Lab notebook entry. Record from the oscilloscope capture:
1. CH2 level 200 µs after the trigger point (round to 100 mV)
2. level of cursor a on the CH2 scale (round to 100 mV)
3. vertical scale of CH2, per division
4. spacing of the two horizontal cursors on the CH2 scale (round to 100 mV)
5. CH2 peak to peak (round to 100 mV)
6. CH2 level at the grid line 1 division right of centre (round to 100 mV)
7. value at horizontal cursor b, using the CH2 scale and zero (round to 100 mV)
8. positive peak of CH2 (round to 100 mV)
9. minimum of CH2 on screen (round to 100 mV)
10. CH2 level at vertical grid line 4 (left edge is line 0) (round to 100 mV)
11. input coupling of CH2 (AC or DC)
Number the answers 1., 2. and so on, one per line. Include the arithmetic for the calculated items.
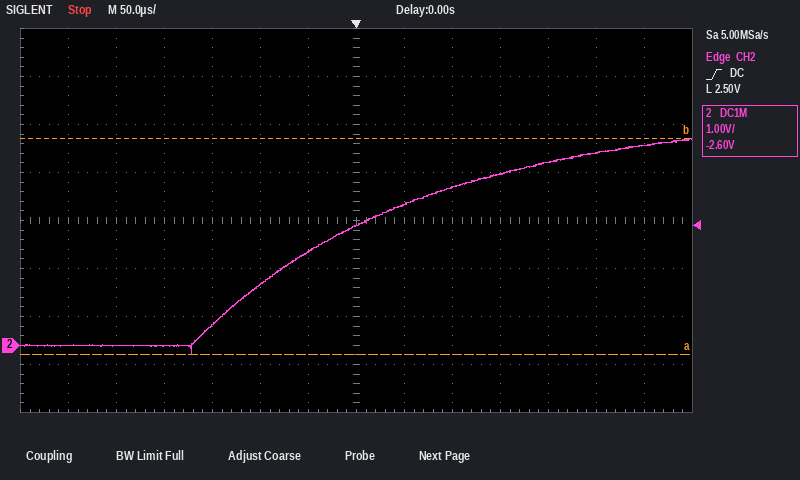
1. 3.8 V
2. -200 mV
3. 1 V
4. 4.5 V
5. 4.3 V − (-200 mV) = 4.5 V
6. 2.9 V
7. 4.3 V
8. 4.3 V
9. -200 mV
10. 400 mV
11. DC
